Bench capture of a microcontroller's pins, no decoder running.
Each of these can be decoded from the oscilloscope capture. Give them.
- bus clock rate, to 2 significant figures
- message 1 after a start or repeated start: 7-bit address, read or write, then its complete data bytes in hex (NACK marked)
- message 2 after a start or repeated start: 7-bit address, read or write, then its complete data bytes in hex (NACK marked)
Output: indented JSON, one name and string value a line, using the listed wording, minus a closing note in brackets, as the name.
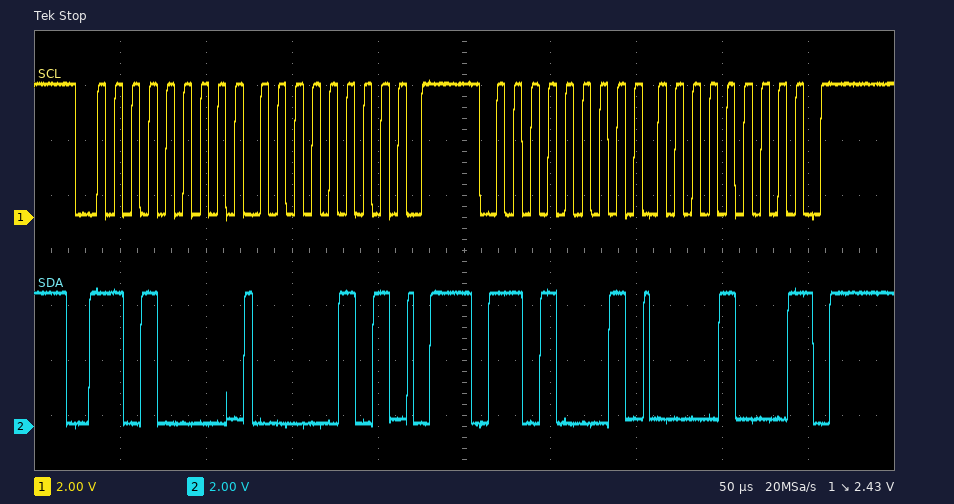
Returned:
{
  "bus clock rate, to 2 significant figures": "100 kHz",
  "message 1 after a start or repeated start: 7-bit address, read or write, then its complete data bytes in hex": "0x68 write: 05",
  "message 2 after a start or repeated start: 7-bit address, read or write, then its complete data bytes in hex": "0x68 read: 08 NACK"
}
